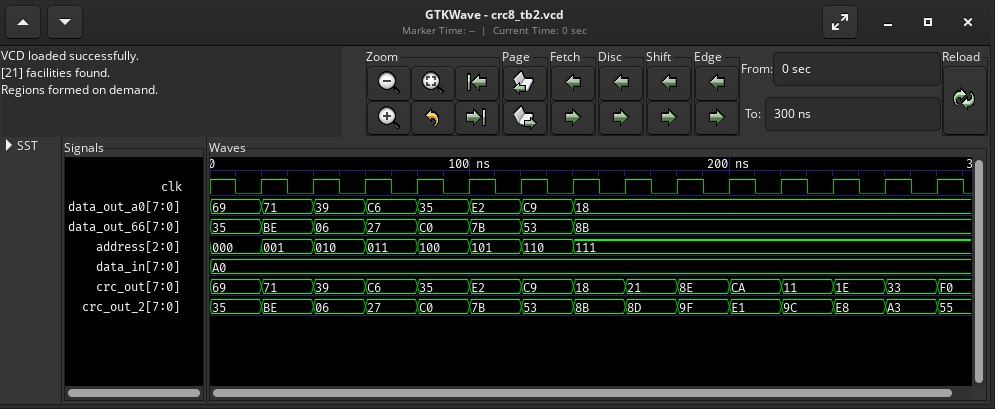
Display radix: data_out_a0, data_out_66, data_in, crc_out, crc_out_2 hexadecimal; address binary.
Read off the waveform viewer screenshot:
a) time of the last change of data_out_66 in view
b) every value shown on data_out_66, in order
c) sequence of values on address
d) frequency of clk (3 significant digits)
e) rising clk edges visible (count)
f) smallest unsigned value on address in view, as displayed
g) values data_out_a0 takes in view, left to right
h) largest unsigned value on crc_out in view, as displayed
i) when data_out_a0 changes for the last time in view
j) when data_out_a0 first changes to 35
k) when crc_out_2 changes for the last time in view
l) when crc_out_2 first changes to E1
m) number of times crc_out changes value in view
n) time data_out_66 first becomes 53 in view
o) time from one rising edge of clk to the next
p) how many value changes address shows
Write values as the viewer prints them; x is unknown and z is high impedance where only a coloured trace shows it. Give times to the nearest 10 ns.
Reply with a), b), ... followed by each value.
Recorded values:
a) 140 ns
b) 35, BE, 06, 27, C0, 7B, 53, 8B
c) 000, 001, 010, 011, 100, 101, 110, 111
d) 50.0 MHz
e) 14
f) 000
g) 69, 71, 39, C6, 35, E2, C9, 18
h) F0
i) 140 ns
j) 80 ns
k) 280 ns
l) 200 ns
m) 14
n) 120 ns
o) 20 ns
p) 7
